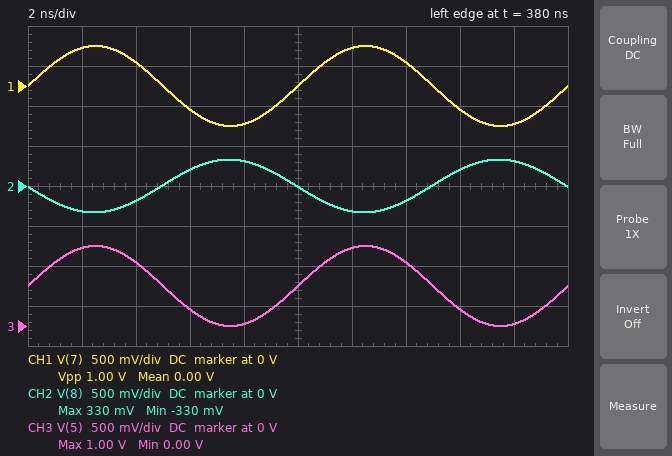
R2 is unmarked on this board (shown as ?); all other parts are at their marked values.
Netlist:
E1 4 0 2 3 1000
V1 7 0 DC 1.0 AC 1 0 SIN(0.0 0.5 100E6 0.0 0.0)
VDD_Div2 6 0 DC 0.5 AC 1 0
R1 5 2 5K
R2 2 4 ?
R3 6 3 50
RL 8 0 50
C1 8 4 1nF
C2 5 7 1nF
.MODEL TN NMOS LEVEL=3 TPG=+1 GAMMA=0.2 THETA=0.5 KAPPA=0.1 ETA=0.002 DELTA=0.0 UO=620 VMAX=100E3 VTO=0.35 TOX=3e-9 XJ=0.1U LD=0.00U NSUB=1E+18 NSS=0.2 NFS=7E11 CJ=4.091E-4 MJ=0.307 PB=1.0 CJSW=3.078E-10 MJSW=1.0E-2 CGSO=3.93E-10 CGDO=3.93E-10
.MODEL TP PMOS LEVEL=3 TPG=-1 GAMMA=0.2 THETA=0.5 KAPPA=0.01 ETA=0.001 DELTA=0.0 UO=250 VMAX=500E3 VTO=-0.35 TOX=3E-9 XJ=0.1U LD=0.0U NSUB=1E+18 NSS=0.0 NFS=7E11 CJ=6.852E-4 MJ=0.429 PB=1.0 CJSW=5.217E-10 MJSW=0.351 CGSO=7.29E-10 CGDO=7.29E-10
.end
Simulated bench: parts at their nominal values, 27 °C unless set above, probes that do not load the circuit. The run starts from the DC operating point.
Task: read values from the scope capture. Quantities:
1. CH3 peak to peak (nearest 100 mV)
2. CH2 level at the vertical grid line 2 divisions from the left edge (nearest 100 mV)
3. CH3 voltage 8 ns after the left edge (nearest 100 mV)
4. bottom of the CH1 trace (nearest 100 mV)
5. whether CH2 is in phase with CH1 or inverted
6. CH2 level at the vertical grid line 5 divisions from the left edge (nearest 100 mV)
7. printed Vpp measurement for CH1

1.0 V
-200 mV
0 V
-500 mV
inverted
0 V
1.00 V
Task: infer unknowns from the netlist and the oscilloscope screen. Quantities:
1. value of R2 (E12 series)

3.3 kΩ
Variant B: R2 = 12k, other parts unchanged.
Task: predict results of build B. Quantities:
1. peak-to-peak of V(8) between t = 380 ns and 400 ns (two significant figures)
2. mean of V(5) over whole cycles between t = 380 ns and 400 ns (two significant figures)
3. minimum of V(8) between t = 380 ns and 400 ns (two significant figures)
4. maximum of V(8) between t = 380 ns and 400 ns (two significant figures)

2.4 V
500 mV
-1.2 V
1.2 V
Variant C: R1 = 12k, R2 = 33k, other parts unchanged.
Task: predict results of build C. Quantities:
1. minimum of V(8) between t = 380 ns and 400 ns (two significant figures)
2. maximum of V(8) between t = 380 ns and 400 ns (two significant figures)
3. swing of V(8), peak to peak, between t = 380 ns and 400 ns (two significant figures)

-1.4 V
1.4 V
2.8 V
